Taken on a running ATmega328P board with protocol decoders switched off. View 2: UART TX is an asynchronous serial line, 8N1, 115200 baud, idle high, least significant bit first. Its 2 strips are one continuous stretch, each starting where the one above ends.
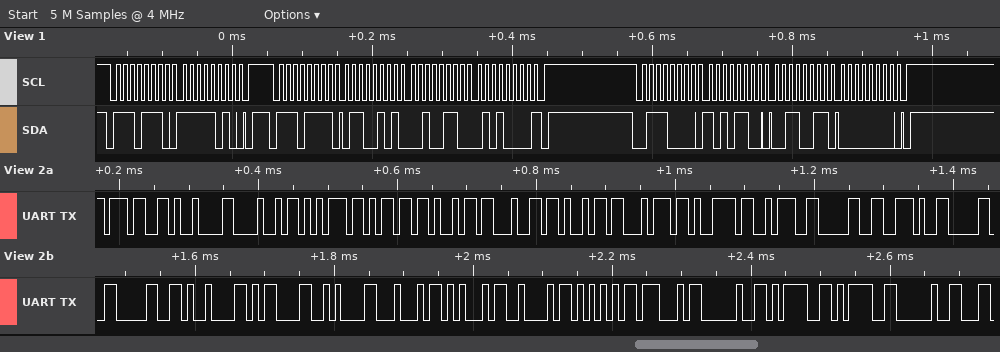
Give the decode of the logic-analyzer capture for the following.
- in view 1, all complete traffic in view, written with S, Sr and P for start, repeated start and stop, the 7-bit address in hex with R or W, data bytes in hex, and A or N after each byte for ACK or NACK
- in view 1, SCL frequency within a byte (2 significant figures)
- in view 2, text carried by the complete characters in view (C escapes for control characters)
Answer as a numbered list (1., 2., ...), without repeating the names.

1. S 77W A FA A P S 77R A 65 A 26 A 50 N P S 38W A AC A 33 A 00 A P
2. 100 kHz
3. "7\tHumidity:0.00\t\r\nDEBUG == "
